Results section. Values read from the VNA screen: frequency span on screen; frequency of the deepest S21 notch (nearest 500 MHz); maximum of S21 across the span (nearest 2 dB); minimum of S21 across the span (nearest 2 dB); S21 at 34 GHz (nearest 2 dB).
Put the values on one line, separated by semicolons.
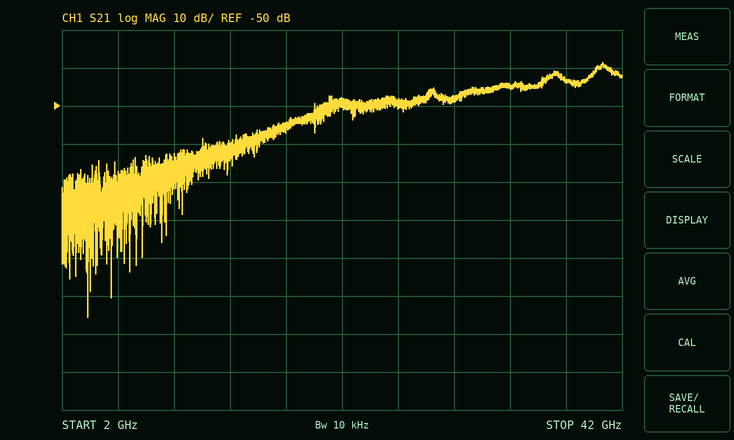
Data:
40 GHz; 4.0 GHz; -38 dB; -106 dB; -44 dB
